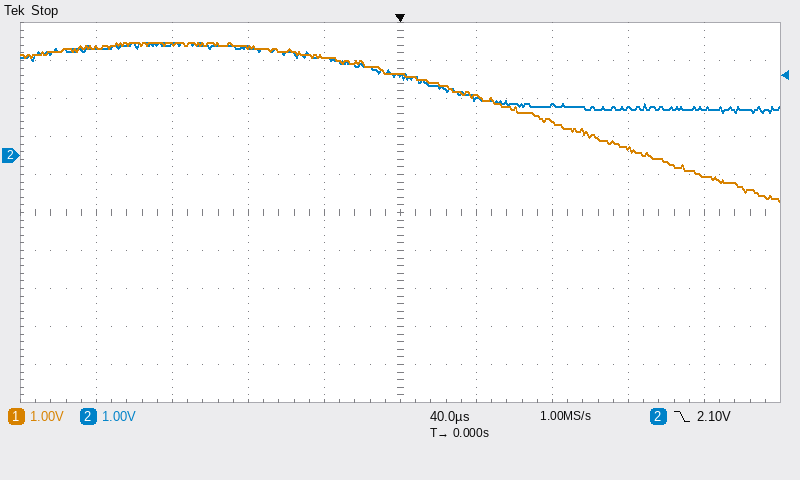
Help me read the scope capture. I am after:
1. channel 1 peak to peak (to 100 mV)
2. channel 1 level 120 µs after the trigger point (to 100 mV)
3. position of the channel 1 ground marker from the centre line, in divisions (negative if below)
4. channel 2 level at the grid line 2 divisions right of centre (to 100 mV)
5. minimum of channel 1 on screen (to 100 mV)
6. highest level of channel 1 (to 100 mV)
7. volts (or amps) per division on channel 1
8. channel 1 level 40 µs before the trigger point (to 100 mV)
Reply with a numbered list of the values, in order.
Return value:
1. 4.2 V
2. 200 mV
3. +1.5 div
4. 1.3 V
5. -1.2 V
6. 3.0 V
7. 1 V
8. 2.6 V
